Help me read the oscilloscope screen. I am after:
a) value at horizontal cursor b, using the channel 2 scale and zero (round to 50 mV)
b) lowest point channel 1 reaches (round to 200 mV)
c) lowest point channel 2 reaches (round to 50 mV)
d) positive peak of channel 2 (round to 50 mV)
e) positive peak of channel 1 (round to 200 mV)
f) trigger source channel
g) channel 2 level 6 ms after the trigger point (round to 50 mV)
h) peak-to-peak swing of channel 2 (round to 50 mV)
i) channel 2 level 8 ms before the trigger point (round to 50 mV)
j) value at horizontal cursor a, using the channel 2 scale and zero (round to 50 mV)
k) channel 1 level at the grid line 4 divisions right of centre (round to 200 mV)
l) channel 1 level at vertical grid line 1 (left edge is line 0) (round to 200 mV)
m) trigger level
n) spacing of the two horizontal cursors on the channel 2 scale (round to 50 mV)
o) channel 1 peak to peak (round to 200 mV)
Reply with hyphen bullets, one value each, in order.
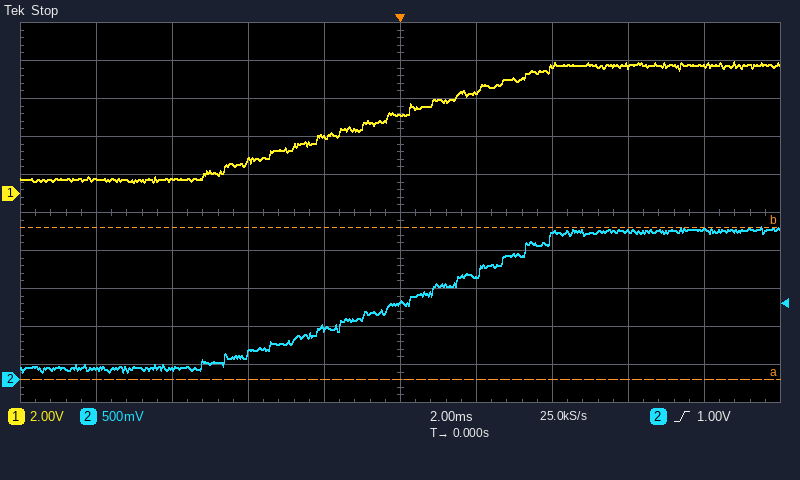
- 2.00 V
- 600 mV
- 100 mV
- 2.00 V
- 7.0 V
- channel 2
- 1.95 V
- 1.90 V
- 150 mV
- 0 mV
- 6.8 V
- 800 mV
- 1.00 V
- 2.00 V
- 6.4 V
